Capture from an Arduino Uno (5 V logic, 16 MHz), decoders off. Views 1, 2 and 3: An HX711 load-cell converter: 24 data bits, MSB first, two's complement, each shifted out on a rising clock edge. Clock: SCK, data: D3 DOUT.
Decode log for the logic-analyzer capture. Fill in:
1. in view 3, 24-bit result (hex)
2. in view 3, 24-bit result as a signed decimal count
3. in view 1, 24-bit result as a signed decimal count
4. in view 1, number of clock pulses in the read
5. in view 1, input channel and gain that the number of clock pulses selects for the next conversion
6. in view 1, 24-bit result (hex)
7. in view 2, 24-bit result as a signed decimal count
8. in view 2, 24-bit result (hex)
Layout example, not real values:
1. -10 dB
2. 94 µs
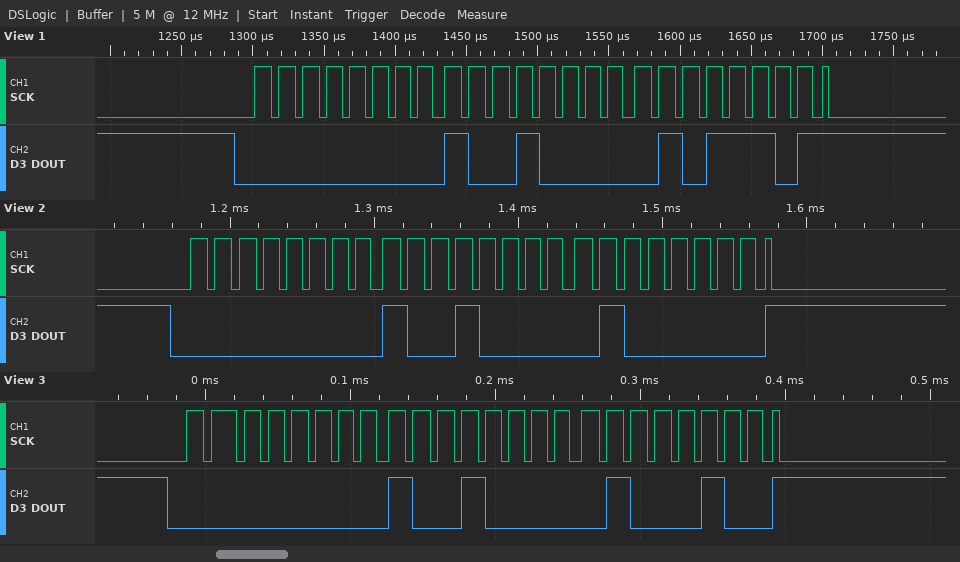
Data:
1. 0x009044
2. 36932
3. 36957
4. 25
5. channel A, gain 128
6. 0x00905D
7. 36928
8. 0x009040
